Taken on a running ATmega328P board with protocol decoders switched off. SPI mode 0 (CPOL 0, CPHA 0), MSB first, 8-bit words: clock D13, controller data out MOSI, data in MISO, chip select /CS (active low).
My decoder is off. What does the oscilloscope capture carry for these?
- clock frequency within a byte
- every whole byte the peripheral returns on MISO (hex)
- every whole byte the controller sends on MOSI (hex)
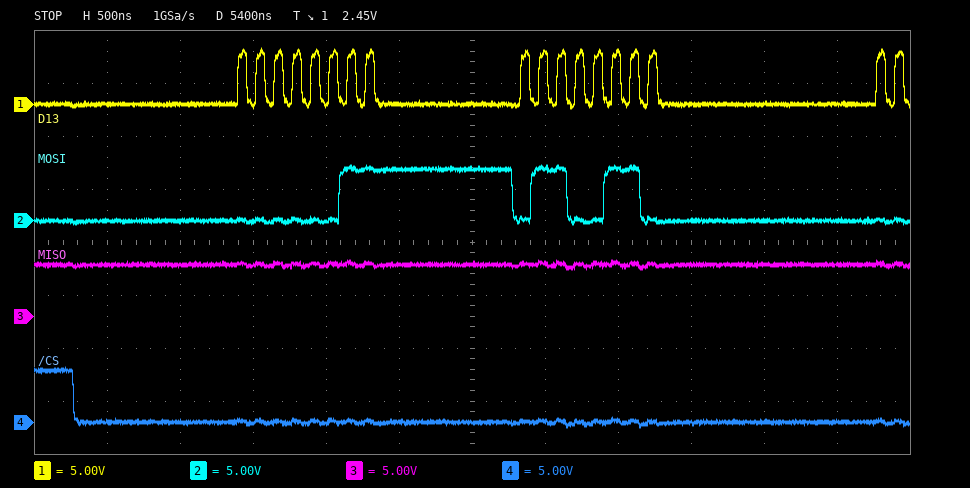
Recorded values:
8 MHz
FF FF
03 66
